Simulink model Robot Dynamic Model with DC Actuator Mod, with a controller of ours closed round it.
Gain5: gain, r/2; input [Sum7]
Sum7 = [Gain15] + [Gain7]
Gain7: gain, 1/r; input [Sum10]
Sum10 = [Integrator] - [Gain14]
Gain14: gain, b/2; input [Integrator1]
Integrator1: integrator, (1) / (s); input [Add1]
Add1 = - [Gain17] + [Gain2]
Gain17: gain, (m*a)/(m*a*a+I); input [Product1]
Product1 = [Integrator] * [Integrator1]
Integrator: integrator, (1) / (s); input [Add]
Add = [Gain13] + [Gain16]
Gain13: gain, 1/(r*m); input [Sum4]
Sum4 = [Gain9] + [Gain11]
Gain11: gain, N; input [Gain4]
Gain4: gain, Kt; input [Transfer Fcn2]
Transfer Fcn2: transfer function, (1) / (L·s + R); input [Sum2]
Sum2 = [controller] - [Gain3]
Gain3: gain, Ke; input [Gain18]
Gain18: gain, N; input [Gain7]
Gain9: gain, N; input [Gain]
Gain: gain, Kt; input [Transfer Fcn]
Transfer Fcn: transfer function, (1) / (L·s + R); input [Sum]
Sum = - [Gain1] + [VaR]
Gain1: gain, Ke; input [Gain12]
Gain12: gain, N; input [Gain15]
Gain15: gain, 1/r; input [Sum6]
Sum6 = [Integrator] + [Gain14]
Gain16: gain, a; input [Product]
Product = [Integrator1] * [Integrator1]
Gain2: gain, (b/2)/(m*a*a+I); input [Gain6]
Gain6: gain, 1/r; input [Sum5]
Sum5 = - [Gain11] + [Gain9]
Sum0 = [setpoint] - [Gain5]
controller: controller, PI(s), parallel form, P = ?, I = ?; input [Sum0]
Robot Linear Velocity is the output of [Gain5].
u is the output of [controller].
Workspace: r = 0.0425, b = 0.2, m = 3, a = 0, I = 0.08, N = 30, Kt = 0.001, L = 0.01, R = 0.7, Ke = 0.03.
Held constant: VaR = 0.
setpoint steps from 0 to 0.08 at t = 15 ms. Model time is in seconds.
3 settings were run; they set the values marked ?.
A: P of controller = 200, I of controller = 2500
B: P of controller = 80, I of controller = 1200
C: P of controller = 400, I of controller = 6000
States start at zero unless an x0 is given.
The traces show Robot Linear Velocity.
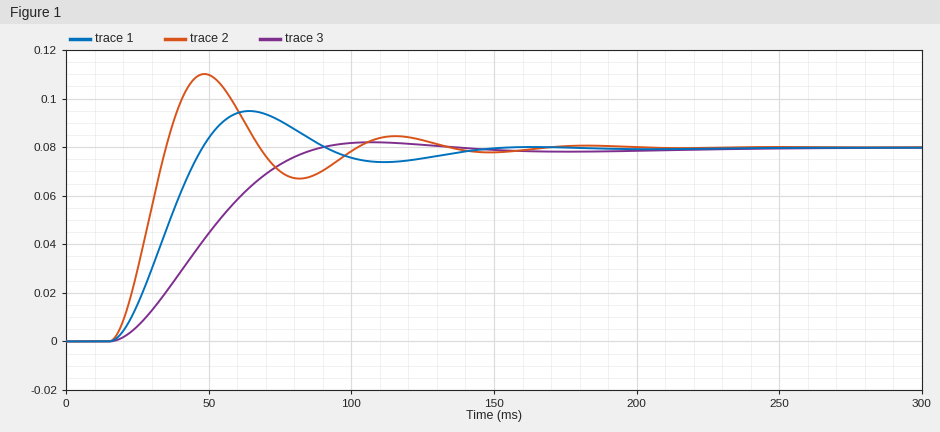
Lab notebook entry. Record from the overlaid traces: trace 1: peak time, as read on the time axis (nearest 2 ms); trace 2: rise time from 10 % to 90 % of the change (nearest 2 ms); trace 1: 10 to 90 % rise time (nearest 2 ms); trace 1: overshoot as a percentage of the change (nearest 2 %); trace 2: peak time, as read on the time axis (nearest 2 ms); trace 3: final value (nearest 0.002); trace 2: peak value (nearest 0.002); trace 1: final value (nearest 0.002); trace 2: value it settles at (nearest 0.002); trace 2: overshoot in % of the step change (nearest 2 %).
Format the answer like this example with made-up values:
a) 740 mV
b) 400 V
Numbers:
a) 64 ms
b) 14 ms
c) 22 ms
d) 18 %
e) 48 ms
f) 0.080
g) 0.110
h) 0.080
i) 0.080
j) 38 %
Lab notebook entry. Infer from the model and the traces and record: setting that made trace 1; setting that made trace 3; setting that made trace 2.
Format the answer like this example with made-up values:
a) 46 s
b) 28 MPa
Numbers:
a) A
b) B
c) C
